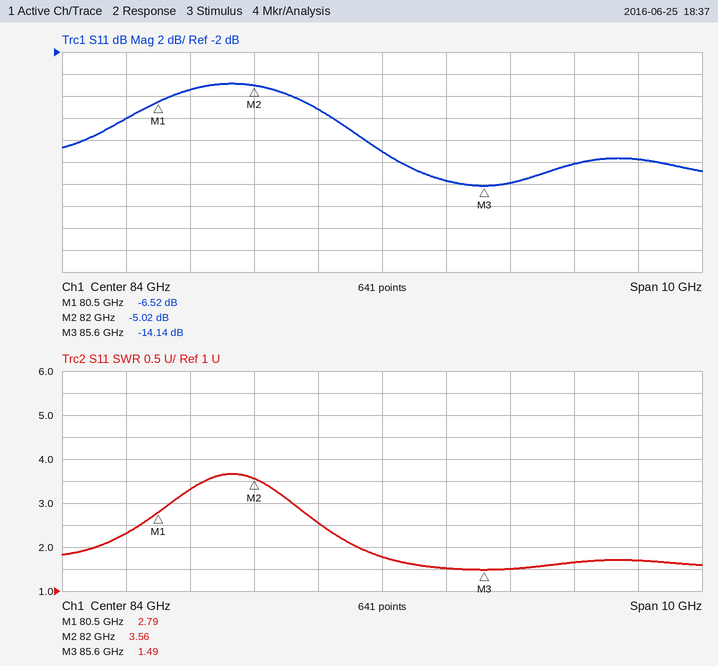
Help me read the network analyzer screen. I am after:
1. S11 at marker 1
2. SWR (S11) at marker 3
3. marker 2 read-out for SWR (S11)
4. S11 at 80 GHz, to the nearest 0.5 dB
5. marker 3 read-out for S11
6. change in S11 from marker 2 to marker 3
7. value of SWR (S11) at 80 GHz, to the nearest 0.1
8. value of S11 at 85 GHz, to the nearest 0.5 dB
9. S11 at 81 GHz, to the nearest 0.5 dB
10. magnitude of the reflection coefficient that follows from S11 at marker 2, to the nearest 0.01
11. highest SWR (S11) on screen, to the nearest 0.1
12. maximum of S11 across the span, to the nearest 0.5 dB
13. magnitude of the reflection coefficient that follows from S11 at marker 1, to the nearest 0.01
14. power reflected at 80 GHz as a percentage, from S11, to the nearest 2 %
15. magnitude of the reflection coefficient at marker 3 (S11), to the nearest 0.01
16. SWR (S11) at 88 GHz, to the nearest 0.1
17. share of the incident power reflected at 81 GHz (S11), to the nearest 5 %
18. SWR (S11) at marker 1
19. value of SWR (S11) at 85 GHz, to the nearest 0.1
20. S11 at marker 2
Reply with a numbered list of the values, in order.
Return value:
1. -6.52 dB
2. 1.49
3. 3.56
4. -8.0 dB
5. -14.14 dB
6. -9.12 dB
7. 2.3
8. -13.5 dB
9. -5.5 dB
10. 0.56
11. 3.7
12. -5.0 dB
13. 0.47
14. 16 %
15. 0.20
16. 1.7
17. 30 %
18. 2.79
19. 1.5
20. -5.02 dB
